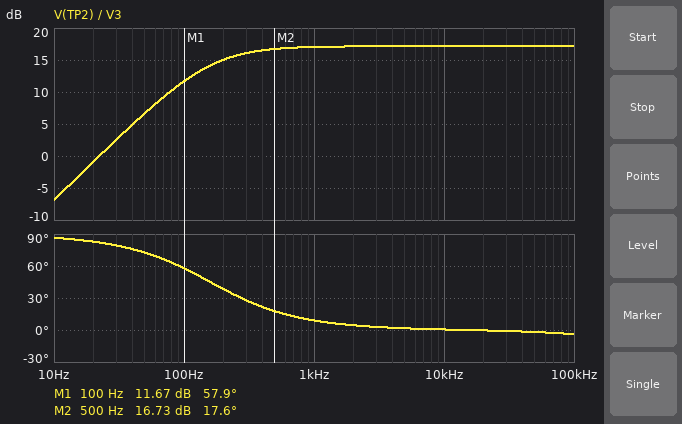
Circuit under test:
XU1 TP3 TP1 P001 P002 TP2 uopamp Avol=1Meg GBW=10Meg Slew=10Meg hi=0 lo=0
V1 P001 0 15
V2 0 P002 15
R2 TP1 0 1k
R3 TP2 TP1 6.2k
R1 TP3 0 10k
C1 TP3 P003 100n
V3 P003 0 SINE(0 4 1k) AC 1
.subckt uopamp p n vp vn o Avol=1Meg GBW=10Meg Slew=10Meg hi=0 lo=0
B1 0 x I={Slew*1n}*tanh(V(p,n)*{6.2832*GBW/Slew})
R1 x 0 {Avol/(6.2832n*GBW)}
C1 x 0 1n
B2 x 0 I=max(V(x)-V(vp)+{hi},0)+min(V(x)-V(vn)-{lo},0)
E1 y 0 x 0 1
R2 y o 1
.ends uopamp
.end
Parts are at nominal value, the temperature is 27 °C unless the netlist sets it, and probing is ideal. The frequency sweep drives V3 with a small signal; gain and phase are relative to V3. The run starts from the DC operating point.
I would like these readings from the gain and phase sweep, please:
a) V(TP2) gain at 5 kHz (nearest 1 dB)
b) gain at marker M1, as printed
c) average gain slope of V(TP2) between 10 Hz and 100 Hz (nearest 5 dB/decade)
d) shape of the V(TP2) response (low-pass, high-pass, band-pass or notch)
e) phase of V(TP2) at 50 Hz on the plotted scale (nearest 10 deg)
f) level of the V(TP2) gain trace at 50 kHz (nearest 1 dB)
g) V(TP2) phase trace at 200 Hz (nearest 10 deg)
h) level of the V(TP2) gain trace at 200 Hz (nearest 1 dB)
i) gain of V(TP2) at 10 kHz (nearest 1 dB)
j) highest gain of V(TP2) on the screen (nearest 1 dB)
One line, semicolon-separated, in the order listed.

17 dB; 11.67 dB; 20 dB/decade; high-pass; 70 deg; 17 dB; 40 deg; 15 dB; 17 dB; 17 dB
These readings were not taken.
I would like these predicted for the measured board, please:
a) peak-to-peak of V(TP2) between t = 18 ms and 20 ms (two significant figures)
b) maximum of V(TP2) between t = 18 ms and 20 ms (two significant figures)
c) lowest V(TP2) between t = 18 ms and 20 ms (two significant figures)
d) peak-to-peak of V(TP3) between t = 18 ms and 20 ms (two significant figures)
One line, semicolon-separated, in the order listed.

30 V; 15 V; -15 V; 7.9 V
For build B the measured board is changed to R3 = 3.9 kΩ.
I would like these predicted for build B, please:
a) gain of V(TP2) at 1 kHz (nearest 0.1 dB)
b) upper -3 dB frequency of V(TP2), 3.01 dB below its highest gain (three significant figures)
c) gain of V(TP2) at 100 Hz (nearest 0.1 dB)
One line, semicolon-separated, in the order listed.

13.7 dB; 2.04 MHz; 8.3 dB
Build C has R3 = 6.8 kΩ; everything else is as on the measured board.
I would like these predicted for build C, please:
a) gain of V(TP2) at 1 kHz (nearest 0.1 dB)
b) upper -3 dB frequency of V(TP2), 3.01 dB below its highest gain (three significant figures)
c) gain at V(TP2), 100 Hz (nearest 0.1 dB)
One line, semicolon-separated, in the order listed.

17.7 dB; 1.28 MHz; 12.4 dB
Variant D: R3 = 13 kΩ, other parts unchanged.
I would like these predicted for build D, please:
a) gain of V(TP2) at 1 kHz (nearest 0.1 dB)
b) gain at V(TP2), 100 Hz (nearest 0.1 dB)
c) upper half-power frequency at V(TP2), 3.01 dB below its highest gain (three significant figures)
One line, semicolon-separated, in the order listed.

22.8 dB; 17.4 dB; 715 kHz
